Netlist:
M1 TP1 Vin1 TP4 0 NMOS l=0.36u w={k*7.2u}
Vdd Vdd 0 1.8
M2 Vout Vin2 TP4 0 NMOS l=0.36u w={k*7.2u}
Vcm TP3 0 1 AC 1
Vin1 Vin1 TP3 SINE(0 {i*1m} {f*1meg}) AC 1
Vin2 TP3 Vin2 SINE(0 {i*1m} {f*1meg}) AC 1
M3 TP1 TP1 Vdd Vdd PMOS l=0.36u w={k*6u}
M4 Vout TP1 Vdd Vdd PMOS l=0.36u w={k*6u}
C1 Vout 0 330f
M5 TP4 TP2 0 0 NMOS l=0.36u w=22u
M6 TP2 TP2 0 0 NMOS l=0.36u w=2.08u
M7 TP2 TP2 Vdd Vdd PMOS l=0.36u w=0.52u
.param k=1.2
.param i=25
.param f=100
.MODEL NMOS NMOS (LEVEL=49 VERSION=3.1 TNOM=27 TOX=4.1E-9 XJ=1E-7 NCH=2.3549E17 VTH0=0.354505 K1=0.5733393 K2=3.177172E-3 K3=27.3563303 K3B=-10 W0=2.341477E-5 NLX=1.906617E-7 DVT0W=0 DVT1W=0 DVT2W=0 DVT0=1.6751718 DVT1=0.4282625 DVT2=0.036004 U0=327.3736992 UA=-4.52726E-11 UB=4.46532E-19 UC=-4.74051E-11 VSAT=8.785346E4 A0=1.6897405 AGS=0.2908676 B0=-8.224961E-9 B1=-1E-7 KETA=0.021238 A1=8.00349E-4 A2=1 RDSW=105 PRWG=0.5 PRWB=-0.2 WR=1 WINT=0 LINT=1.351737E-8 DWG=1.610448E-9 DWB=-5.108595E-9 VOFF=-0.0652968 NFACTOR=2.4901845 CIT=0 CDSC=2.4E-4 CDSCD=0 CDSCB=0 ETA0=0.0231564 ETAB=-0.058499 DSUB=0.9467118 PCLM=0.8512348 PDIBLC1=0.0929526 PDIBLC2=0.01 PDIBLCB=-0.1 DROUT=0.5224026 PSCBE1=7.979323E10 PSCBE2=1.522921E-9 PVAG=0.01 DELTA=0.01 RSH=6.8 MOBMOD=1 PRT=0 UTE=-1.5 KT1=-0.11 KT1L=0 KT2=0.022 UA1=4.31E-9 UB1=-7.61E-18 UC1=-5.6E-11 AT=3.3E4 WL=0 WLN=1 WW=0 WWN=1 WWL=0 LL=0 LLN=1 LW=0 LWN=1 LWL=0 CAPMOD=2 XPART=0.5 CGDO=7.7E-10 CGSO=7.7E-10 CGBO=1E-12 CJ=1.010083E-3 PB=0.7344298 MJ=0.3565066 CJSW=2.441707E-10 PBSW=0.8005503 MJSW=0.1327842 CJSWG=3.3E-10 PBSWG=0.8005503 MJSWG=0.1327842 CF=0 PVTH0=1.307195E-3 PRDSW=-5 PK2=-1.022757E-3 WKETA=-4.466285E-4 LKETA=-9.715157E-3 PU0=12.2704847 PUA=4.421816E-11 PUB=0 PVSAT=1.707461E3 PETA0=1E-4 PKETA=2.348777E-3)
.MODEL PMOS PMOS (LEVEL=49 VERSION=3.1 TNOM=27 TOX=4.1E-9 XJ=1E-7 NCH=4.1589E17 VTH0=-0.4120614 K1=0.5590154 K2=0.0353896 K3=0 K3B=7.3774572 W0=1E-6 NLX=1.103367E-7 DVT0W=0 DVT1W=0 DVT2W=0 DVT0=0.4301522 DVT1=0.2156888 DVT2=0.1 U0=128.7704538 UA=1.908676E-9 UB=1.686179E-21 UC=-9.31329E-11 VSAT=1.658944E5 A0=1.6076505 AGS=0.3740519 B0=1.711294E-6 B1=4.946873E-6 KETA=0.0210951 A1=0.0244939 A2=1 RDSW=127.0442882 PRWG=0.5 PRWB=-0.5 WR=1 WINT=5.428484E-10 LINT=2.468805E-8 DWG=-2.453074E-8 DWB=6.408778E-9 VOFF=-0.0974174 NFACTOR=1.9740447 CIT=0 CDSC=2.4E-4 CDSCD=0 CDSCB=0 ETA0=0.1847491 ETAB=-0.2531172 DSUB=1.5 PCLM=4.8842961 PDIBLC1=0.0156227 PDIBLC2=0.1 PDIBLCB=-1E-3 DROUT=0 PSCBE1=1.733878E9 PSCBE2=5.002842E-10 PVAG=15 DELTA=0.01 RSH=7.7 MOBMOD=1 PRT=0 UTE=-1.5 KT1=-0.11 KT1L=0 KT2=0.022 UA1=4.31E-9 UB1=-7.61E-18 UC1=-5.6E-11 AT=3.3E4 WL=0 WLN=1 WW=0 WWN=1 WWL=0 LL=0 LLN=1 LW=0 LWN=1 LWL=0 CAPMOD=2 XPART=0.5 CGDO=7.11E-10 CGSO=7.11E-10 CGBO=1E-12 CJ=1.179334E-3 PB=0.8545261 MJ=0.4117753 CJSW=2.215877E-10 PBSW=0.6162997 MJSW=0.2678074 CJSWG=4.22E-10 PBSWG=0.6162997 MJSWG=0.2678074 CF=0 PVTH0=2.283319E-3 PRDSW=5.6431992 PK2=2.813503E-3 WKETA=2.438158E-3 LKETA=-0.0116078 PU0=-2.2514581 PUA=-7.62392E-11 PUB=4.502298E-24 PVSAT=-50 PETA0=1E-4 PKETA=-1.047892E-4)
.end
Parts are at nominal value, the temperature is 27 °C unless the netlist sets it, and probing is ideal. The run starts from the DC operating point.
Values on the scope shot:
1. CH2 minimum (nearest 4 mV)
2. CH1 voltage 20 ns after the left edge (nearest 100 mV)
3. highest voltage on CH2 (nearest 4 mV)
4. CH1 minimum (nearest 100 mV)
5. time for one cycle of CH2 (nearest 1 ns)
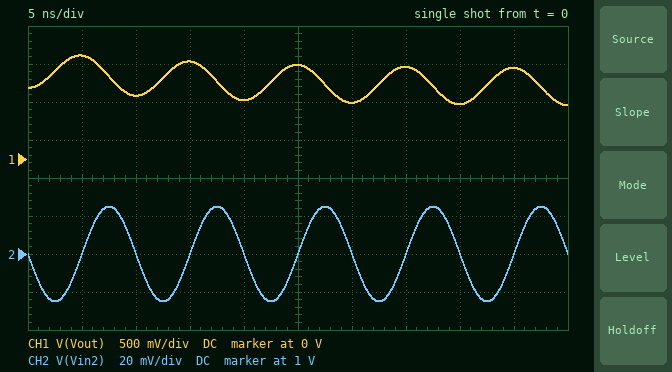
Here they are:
976 mV
800 mV
1.024 V
700 mV
10 ns
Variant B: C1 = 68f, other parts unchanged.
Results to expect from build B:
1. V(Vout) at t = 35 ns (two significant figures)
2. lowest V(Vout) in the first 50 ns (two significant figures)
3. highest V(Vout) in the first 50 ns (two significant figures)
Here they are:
1.5 V
350 mV
1.6 V
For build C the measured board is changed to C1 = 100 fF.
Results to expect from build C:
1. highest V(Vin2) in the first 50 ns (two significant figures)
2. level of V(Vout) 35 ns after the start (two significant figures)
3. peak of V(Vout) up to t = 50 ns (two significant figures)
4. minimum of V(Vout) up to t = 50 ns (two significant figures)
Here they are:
1.0 V
1.5 V
1.6 V
370 mV
